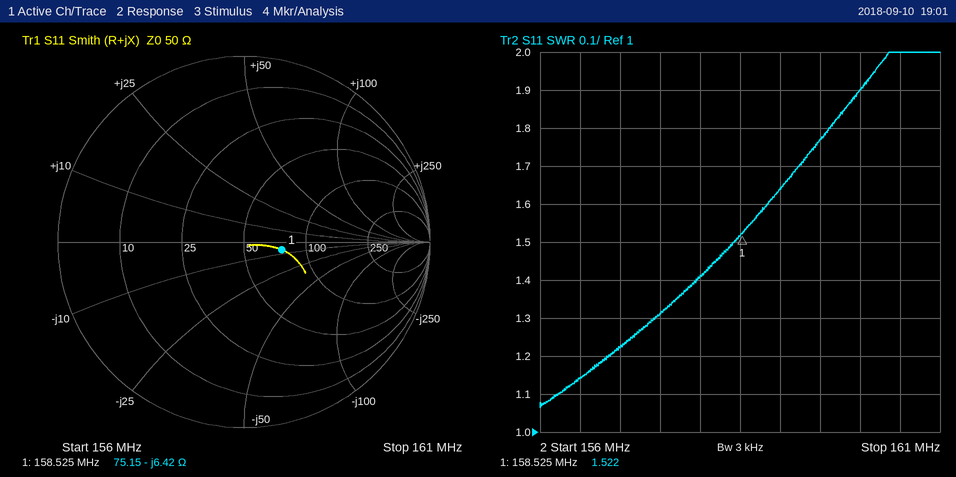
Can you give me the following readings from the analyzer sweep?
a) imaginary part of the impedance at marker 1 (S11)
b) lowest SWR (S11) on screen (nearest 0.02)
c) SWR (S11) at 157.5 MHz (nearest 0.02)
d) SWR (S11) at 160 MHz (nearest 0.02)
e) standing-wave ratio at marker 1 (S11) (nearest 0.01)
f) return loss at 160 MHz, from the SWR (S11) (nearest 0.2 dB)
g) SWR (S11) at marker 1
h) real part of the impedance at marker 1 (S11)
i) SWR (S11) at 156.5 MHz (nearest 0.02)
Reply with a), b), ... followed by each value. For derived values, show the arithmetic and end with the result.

a) -6.42 Ω
b) 1.06
c) 1.32
d) 1.90
e) 1.52
f) −20 log10((1.9 − 1)/(1.9 + 1)) ≈ 10.2 dB
g) 1.522
h) 75.15 Ω
i) 1.14
